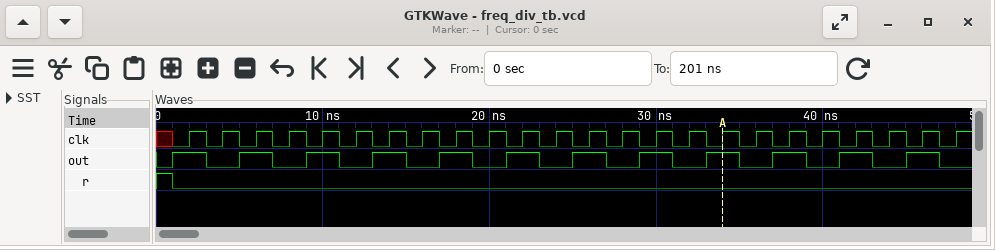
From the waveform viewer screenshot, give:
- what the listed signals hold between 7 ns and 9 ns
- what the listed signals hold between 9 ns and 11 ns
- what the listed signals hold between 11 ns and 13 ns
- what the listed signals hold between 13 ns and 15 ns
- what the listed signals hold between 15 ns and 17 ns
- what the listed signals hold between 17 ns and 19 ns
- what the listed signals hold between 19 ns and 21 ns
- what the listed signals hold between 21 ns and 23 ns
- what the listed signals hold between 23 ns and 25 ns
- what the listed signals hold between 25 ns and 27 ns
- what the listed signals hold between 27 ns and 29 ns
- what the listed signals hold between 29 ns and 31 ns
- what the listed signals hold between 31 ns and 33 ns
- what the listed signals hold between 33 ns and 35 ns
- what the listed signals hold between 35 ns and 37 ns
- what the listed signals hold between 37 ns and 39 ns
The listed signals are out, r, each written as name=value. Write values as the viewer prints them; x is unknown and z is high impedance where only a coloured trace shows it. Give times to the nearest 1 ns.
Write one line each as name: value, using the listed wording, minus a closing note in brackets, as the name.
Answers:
what the listed signals hold between 7 ns and 9 ns: out=0, r=0
what the listed signals hold between 9 ns and 11 ns: out=1, r=0
what the listed signals hold between 11 ns and 13 ns: out=0, r=0
what the listed signals hold between 13 ns and 15 ns: out=1, r=0
what the listed signals hold between 15 ns and 17 ns: out=0, r=0
what the listed signals hold between 17 ns and 19 ns: out=1, r=0
what the listed signals hold between 19 ns and 21 ns: out=0, r=0
what the listed signals hold between 21 ns and 23 ns: out=1, r=0
what the listed signals hold between 23 ns and 25 ns: out=0, r=0
what the listed signals hold between 25 ns and 27 ns: out=1, r=0
what the listed signals hold between 27 ns and 29 ns: out=0, r=0
what the listed signals hold between 29 ns and 31 ns: out=1, r=0
what the listed signals hold between 31 ns and 33 ns: out=0, r=0
what the listed signals hold between 33 ns and 35 ns: out=1, r=0
what the listed signals hold between 35 ns and 37 ns: out=0, r=0
what the listed signals hold between 37 ns and 39 ns: out=1, r=0
